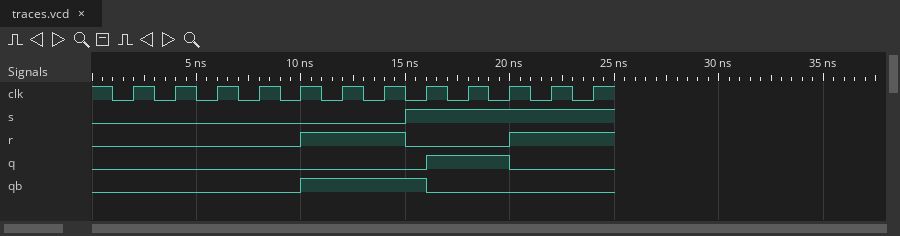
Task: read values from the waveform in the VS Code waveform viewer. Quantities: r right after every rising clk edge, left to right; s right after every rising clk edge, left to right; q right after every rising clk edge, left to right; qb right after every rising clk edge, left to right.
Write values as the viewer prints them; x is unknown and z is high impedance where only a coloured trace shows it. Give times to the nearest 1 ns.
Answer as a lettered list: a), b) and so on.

a) 0 0 0 0 1 1 1 0 0 1 1 1
b) 0 0 0 0 0 0 0 1 1 1 1 1
c) 0 0 0 0 0 0 0 1 1 0 0 0
d) 0 0 0 0 1 1 1 0 0 0 0 0
